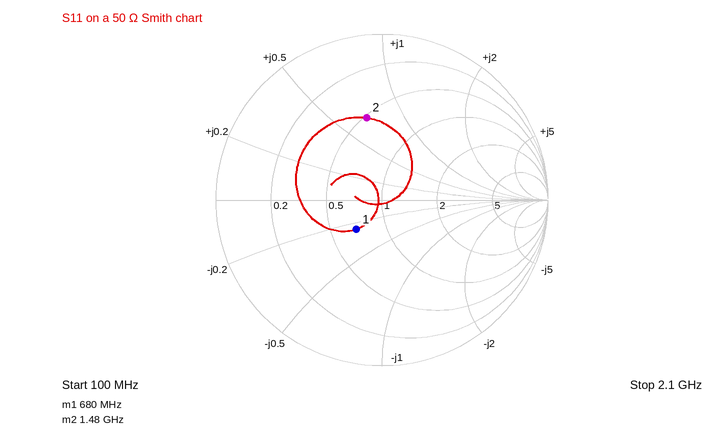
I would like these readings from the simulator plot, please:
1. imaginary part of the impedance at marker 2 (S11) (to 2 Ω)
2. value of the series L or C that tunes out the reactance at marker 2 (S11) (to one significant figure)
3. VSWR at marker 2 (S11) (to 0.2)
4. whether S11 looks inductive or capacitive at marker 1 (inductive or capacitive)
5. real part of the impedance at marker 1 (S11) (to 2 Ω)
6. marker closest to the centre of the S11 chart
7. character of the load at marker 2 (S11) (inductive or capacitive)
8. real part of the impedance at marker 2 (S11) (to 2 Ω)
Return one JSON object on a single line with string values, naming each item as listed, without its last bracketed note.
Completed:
{"imaginary part of the impedance at marker 2 (S11)": "+34 Ω", "value of the series L or C that tunes out the reactance at marker 2 (S11)": "3 pF", "VSWR at marker 2 (S11)": "3.0", "whether S11 looks inductive or capacitive at marker 1": "capacitive", "real part of the impedance at marker 1 (S11)": "34 Ω", "marker closest to the centre of the S11 chart": "marker 1", "character of the load at marker 2 (S11)": "inductive", "real part of the impedance at marker 2 (S11)": "26 Ω"}
